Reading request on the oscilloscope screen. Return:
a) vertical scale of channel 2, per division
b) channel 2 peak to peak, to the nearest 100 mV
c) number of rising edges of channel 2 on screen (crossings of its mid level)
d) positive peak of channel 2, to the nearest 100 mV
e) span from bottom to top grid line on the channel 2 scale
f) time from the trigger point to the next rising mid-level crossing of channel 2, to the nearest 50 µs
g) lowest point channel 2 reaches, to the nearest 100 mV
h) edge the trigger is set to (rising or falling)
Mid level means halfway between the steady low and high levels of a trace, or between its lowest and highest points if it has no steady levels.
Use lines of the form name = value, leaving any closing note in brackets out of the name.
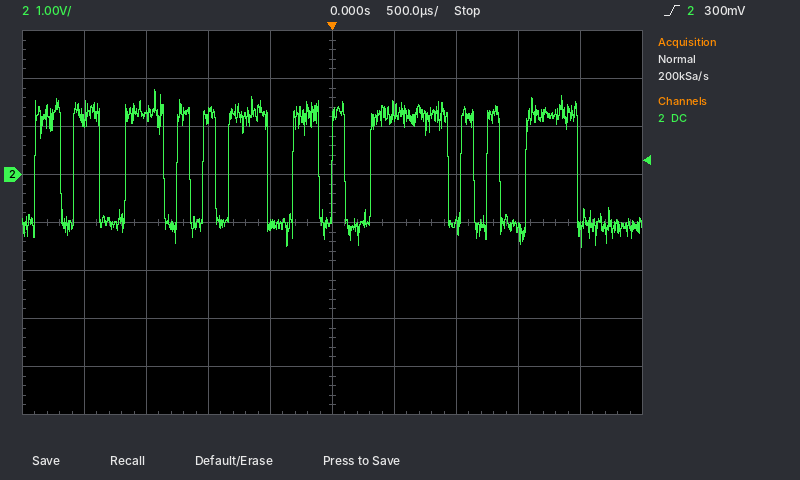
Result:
vertical scale of channel 2, per division = 1 V
channel 2 peak to peak, to the nearest 100 mV = 3.3 V
number of rising edges of channel 2 on screen = 12
positive peak of channel 2, to the nearest 100 mV = 1.8 V
span from bottom to top grid line on the channel 2 scale = 8 V
time from the trigger point to the next rising mid-level crossing of channel 2, to the nearest 50 µs = 300 µs
lowest point channel 2 reaches, to the nearest 100 mV = -1.5 V
edge the trigger is set to = rising
